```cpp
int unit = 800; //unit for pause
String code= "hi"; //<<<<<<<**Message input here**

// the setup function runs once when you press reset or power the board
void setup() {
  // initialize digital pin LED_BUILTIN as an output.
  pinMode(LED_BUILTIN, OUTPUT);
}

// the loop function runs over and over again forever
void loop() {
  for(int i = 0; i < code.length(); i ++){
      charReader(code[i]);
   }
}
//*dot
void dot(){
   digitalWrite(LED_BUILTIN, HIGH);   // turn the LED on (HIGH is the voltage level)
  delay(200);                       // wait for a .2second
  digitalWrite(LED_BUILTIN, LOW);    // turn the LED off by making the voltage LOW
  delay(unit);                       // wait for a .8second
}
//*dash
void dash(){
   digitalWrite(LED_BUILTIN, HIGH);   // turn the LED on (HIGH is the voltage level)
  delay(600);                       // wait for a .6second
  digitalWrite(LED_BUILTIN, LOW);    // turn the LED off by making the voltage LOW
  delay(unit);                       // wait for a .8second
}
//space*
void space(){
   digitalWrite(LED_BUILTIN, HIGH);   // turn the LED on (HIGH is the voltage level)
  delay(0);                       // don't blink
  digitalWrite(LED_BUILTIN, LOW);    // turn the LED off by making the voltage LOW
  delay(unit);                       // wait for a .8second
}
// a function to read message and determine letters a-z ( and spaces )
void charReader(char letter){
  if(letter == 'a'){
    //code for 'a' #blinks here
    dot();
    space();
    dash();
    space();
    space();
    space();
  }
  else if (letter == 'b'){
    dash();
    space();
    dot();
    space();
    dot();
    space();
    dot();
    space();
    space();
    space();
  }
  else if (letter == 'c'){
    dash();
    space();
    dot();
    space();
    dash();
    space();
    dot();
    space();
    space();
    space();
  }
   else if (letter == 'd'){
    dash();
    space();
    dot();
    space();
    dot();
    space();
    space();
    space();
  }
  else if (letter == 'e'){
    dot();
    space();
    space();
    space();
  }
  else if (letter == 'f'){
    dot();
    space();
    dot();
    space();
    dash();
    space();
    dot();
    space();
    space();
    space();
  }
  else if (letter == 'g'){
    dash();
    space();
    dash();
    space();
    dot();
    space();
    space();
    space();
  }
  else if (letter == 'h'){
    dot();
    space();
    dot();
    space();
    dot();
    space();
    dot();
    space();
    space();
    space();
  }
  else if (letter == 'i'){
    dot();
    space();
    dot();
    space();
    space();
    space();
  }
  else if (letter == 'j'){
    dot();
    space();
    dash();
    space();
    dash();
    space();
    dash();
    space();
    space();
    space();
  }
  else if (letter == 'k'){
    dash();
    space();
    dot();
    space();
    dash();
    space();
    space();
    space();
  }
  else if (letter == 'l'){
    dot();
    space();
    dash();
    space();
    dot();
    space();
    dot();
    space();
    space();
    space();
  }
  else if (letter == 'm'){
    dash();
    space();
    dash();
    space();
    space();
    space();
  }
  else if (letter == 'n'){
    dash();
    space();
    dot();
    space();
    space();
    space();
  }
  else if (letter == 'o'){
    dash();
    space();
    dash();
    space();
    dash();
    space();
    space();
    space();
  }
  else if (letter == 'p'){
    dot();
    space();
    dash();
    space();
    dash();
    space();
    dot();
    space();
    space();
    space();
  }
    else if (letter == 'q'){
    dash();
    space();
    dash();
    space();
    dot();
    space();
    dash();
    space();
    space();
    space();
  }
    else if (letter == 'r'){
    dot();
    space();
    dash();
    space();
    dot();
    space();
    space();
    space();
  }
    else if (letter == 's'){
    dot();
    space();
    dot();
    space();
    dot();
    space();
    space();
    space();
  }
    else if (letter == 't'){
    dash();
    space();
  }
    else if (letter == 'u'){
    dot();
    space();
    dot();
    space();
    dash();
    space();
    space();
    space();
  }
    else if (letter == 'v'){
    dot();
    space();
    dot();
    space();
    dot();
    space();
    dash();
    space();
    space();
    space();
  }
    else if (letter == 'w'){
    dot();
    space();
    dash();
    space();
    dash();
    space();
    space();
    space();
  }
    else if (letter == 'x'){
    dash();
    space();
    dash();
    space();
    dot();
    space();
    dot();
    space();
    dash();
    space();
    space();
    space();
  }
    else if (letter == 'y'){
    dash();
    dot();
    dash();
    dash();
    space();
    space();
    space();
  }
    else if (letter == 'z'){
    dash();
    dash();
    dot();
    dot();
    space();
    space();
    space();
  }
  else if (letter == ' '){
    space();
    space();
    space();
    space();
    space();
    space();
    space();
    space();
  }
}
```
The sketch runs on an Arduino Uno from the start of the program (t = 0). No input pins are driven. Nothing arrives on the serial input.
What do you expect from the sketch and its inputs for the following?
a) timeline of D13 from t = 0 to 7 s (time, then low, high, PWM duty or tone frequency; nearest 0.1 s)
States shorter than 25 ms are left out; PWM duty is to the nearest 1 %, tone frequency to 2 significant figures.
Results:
0 s high; 0.2 s low; 1.8 s high; 2 s low; 3.6 s high; 3.8 s low; 5.4 s high; 5.6 s low
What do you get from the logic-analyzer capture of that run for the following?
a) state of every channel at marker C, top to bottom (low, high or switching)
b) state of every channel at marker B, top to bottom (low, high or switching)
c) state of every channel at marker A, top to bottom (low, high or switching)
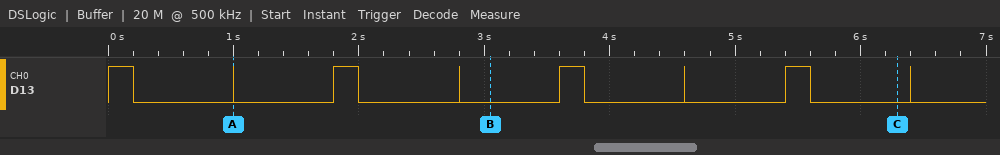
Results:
D13 low
D13 low
D13 low
